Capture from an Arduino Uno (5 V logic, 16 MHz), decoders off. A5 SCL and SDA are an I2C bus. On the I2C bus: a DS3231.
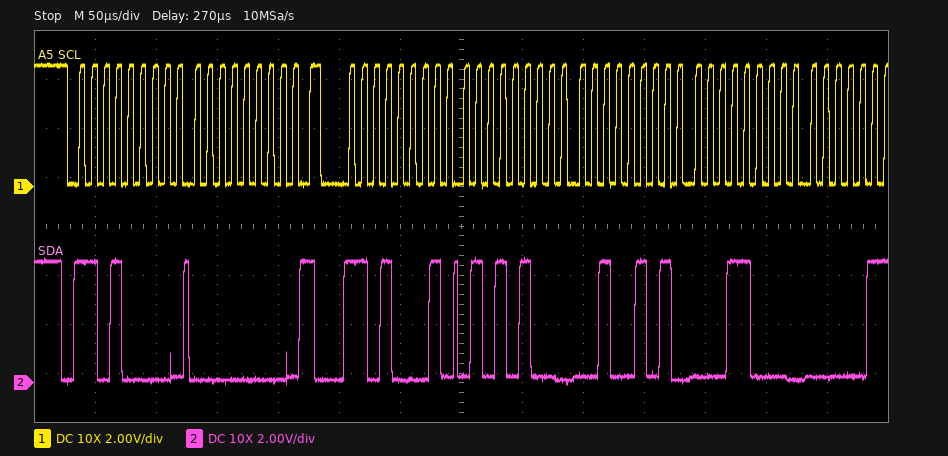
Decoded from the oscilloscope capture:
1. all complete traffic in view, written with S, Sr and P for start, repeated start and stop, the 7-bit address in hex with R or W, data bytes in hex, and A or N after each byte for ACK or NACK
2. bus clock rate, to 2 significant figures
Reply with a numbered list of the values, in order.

1. S 68W A 00 A Sr 68R A 54 A 25 A 18 A
2. 100 kHz
